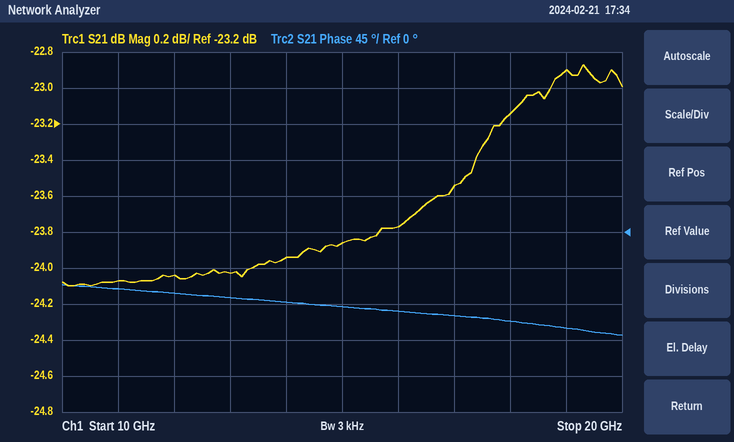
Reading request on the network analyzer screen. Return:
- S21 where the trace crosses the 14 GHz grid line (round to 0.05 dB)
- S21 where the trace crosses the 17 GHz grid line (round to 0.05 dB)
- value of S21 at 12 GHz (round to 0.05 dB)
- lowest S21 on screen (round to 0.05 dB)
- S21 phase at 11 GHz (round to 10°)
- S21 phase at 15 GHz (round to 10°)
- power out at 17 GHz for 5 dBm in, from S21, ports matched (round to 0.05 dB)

-23.95 dB
-23.55 dB
-24.05 dB
-24.10 dB
-70°
-90°
-18.55 dBm
